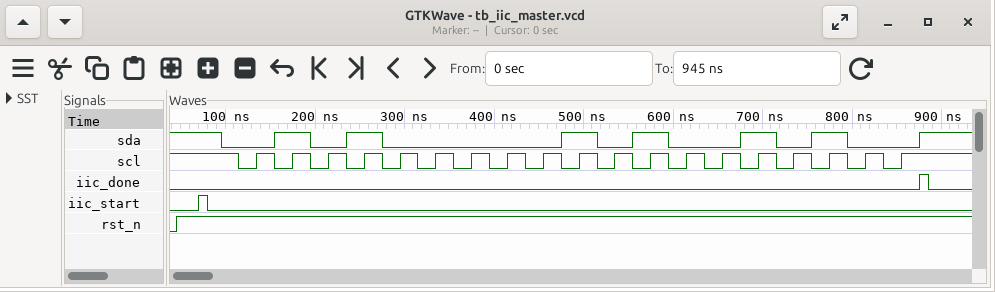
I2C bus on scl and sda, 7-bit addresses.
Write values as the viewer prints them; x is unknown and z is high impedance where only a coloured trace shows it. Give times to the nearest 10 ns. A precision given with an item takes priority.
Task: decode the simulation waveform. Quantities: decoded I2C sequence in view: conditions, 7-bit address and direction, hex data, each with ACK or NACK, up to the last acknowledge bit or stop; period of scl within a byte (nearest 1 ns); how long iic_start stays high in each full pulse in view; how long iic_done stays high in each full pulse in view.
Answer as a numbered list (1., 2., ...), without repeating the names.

1. start, address 28 write ACK, A5 ACK, stop
2. 40 ns
3. 10 ns
4. 10 ns
